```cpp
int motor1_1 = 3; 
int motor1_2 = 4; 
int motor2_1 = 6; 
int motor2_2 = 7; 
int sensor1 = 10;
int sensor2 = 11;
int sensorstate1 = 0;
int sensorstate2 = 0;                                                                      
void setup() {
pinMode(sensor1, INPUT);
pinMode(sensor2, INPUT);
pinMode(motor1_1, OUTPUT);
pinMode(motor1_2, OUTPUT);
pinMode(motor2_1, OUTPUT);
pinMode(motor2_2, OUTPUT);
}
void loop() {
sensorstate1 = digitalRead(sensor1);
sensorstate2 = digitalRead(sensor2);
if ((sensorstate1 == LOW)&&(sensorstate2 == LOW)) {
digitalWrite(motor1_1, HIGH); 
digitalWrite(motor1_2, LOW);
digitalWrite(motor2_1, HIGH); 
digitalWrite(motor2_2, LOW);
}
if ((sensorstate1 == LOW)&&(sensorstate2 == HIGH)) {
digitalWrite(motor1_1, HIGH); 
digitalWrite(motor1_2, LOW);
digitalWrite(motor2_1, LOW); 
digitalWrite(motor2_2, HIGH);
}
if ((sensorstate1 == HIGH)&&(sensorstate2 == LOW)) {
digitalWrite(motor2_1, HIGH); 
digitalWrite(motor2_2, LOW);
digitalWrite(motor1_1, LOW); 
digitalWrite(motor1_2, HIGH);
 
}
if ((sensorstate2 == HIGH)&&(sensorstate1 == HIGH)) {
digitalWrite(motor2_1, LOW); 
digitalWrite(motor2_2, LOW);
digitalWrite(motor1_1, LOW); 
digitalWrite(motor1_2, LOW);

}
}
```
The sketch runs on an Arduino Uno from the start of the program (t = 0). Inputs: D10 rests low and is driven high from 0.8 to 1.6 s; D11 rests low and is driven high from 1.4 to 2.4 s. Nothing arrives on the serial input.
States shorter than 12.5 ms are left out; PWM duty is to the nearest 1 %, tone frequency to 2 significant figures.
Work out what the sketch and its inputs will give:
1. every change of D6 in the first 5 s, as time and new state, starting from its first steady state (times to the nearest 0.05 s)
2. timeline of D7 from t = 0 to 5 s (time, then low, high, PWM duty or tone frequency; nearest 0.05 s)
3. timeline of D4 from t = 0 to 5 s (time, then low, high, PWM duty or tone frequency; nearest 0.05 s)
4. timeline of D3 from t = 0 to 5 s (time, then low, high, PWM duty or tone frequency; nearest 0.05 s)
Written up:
0 s high; 1.4 s low; 2.4 s high
0 s low; 1.6 s high; 2.4 s low
0 s low; 0.8 s high; 1.4 s low
0 s high; 0.8 s low; 1.6 s high
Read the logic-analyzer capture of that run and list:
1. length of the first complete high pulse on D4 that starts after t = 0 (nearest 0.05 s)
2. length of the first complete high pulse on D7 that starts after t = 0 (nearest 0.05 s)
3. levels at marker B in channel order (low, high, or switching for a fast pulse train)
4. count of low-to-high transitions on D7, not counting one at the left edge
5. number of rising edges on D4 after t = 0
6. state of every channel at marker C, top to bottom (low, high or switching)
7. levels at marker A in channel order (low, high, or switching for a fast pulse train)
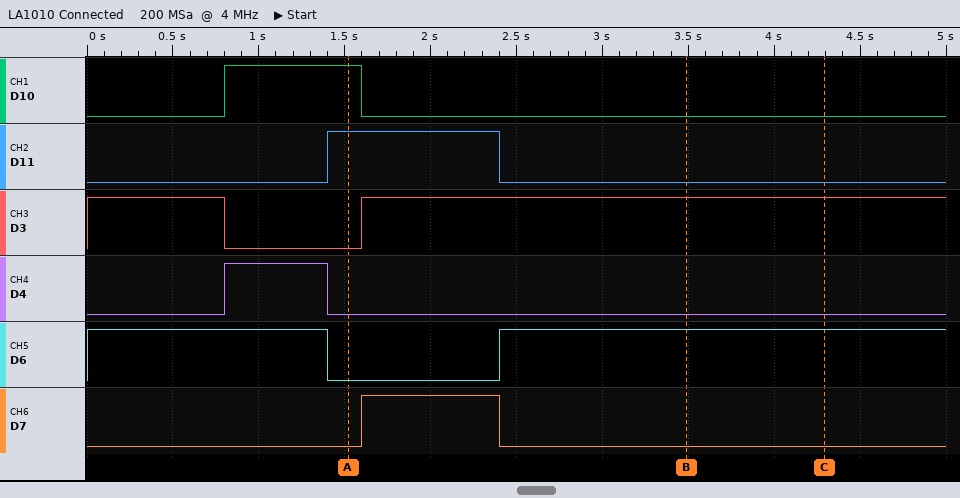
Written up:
0.60 s
0.80 s
D10 low, D11 low, D3 high, D4 low, D6 high, D7 low
1
1
D10 low, D11 low, D3 high, D4 low, D6 high, D7 low
D10 high, D11 high, D3 low, D4 low, D6 low, D7 low
